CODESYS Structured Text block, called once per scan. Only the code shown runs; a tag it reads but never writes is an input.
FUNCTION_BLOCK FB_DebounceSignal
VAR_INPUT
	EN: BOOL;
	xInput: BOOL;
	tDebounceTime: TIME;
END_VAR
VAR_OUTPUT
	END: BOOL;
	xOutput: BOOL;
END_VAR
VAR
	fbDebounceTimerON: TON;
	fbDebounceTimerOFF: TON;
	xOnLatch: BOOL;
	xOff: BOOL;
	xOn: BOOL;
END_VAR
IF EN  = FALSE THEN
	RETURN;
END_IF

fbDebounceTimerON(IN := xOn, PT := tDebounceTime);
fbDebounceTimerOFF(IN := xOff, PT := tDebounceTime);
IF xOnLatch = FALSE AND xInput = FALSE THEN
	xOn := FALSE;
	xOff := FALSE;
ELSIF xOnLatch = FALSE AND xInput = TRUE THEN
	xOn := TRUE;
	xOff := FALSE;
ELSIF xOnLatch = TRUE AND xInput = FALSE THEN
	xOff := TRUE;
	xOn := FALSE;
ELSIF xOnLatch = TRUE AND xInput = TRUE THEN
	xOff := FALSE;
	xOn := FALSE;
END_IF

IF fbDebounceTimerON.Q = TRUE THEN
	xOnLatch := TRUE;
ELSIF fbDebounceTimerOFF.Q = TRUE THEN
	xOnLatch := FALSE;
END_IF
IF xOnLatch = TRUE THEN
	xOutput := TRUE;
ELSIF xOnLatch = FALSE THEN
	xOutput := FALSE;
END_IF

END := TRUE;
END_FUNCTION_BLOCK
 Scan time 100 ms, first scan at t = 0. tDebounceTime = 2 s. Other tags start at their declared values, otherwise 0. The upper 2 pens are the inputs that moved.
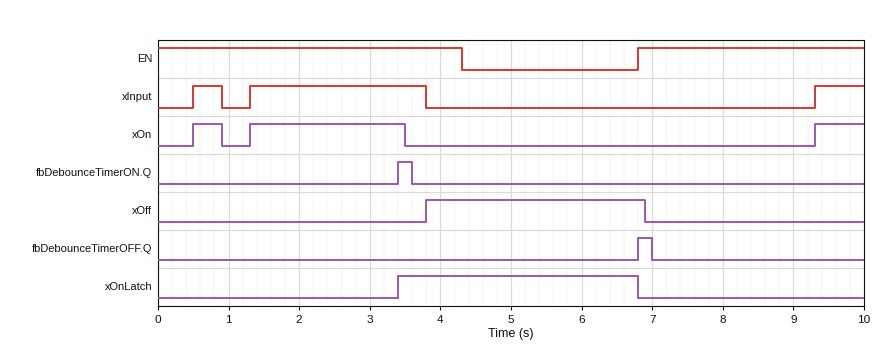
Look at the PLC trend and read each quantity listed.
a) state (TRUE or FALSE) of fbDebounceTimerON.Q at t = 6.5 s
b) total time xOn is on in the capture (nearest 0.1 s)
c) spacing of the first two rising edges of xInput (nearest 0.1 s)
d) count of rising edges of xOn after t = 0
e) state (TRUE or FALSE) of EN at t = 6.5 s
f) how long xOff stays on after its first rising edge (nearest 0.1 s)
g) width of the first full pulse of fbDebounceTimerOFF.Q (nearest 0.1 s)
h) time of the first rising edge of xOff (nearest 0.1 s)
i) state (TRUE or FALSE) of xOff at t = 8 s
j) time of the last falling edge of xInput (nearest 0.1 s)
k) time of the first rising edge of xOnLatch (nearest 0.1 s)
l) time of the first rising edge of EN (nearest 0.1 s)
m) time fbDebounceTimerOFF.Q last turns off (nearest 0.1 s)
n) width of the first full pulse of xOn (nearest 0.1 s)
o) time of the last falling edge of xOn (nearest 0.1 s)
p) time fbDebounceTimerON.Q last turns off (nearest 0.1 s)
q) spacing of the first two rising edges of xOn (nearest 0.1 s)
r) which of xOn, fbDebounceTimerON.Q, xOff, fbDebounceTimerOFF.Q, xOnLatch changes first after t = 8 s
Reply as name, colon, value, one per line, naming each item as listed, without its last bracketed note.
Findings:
state (TRUE or FALSE) of fbDebounceTimerON.Q at t = 6.5 s: FALSE
total time xOn is on in the capture: 3.3 s
spacing of the first two rising edges of xInput: 0.8 s
count of rising edges of xOn after t = 0: 3
state (TRUE or FALSE) of EN at t = 6.5 s: FALSE
how long xOff stays on after its first rising edge: 3.1 s
width of the first full pulse of fbDebounceTimerOFF.Q: 0.2 s
time of the first rising edge of xOff: 3.8 s
state (TRUE or FALSE) of xOff at t = 8 s: FALSE
time of the last falling edge of xInput: 3.8 s
time of the first rising edge of xOnLatch: 3.4 s
time of the first rising edge of EN: 6.8 s
time fbDebounceTimerOFF.Q last turns off: 7.0 s
width of the first full pulse of xOn: 0.4 s
time of the last falling edge of xOn: 3.5 s
time fbDebounceTimerON.Q last turns off: 3.6 s
spacing of the first two rising edges of xOn: 0.8 s
which of xOn, fbDebounceTimerON.Q, xOff, fbDebounceTimerOFF.Q, xOnLatch changes first after t = 8 s: xOn
